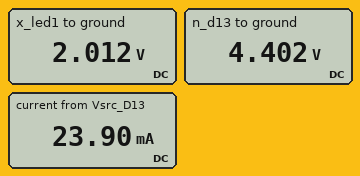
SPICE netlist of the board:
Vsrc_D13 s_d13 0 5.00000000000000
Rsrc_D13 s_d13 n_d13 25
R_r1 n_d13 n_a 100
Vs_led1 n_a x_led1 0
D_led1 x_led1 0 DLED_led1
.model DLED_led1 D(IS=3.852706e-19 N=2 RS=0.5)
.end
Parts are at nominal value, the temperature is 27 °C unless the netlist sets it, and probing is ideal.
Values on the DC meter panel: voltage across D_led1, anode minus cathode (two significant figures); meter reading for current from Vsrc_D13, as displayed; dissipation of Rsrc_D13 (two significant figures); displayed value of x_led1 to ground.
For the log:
2.0 V
23.90 mA
14 mW
2.012 V
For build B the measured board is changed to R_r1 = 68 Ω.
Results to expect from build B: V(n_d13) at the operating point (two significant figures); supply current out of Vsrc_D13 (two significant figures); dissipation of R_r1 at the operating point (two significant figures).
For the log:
4.2 V
32 mA
69 mW
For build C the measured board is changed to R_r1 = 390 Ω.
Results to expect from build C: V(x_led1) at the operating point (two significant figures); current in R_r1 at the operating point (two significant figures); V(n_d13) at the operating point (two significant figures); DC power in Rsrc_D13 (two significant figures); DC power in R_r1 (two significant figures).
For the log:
1.9 V
7.4 mA
4.8 V
1.4 mW
21 mW
